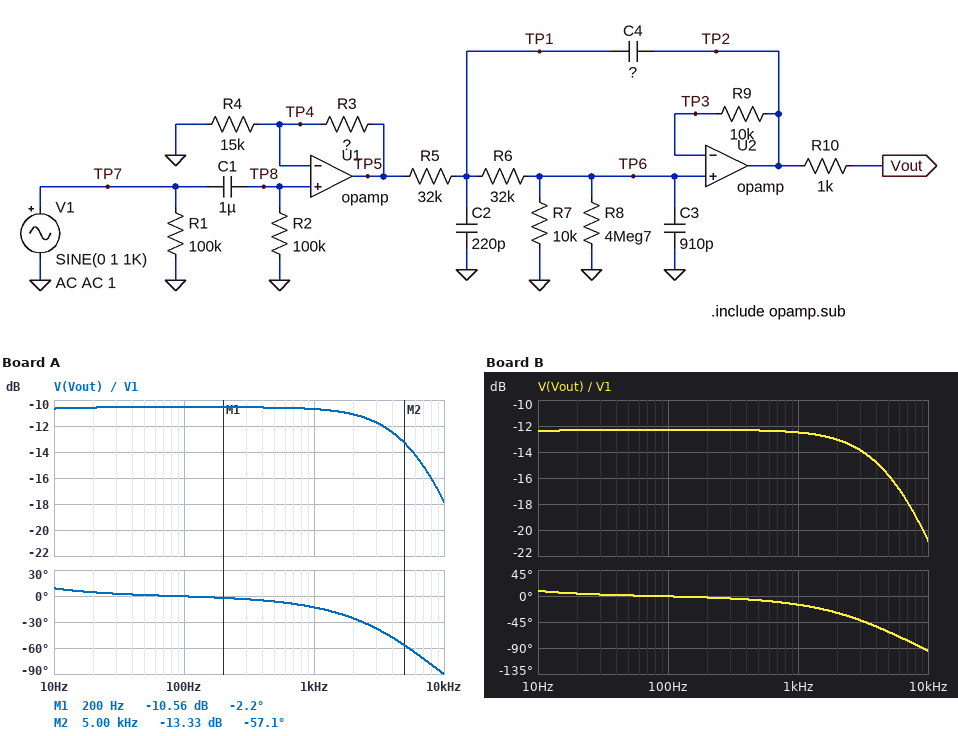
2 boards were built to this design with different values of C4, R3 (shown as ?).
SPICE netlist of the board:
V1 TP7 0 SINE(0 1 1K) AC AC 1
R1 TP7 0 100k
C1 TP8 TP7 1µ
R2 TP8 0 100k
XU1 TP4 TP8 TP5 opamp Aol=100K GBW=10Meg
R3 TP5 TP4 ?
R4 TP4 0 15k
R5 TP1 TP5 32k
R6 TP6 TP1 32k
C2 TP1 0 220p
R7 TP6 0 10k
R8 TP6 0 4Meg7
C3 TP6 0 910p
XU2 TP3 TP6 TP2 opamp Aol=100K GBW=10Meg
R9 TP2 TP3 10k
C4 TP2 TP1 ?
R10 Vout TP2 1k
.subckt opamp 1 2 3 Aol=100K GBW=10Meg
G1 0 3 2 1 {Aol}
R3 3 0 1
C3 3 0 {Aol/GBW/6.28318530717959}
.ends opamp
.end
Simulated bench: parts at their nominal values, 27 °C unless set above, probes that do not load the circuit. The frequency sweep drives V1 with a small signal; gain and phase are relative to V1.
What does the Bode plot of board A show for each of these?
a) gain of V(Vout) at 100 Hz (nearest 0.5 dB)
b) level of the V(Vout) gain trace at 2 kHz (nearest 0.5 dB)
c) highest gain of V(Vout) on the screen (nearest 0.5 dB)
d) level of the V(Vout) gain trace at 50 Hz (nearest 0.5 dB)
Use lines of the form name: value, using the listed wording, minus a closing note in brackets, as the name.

gain of V(Vout) at 100 Hz: -10.5 dB
level of the V(Vout) gain trace at 2 kHz: -11.0 dB
highest gain of V(Vout) on the screen: -10.5 dB
level of the V(Vout) gain trace at 50 Hz: -10.5 dB
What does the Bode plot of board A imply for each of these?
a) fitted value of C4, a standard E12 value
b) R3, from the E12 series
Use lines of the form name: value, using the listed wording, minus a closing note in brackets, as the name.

fitted value of C4, a standard E12 value: 1.8 nF
R3, from the E12 series: 18 kΩ
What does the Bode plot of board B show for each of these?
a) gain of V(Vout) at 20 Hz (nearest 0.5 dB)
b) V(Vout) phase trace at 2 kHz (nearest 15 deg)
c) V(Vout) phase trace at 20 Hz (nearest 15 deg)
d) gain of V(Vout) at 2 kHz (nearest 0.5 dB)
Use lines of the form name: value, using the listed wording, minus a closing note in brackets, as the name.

gain of V(Vout) at 20 Hz: -12.5 dB
V(Vout) phase trace at 2 kHz: -30 deg
V(Vout) phase trace at 20 Hz: 0 deg
gain of V(Vout) at 2 kHz: -13.0 dB
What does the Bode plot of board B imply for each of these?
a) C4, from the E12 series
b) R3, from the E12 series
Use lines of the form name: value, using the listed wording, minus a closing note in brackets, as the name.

C4, from the E12 series: 2.2 nF
R3, from the E12 series: 12 kΩ
